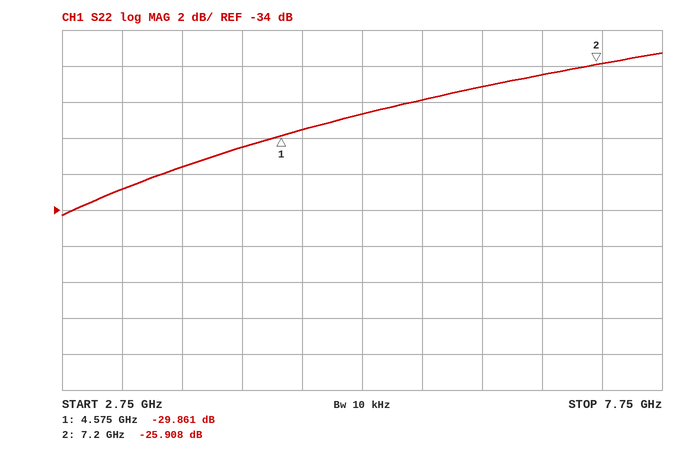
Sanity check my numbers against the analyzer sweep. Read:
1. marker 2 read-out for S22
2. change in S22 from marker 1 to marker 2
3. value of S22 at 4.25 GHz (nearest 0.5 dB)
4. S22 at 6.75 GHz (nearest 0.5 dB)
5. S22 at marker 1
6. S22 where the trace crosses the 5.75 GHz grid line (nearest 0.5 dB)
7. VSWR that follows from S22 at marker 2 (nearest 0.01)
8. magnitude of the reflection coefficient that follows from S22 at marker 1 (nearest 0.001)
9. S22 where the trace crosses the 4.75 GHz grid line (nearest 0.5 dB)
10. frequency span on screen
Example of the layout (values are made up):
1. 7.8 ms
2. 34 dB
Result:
1. -25.908 dB
2. 3.953 dB
3. -30.5 dB
4. -26.5 dB
5. -29.861 dB
6. -28.0 dB
7. 1.11
8. 0.032
9. -29.5 dB
10. 5 GHz
